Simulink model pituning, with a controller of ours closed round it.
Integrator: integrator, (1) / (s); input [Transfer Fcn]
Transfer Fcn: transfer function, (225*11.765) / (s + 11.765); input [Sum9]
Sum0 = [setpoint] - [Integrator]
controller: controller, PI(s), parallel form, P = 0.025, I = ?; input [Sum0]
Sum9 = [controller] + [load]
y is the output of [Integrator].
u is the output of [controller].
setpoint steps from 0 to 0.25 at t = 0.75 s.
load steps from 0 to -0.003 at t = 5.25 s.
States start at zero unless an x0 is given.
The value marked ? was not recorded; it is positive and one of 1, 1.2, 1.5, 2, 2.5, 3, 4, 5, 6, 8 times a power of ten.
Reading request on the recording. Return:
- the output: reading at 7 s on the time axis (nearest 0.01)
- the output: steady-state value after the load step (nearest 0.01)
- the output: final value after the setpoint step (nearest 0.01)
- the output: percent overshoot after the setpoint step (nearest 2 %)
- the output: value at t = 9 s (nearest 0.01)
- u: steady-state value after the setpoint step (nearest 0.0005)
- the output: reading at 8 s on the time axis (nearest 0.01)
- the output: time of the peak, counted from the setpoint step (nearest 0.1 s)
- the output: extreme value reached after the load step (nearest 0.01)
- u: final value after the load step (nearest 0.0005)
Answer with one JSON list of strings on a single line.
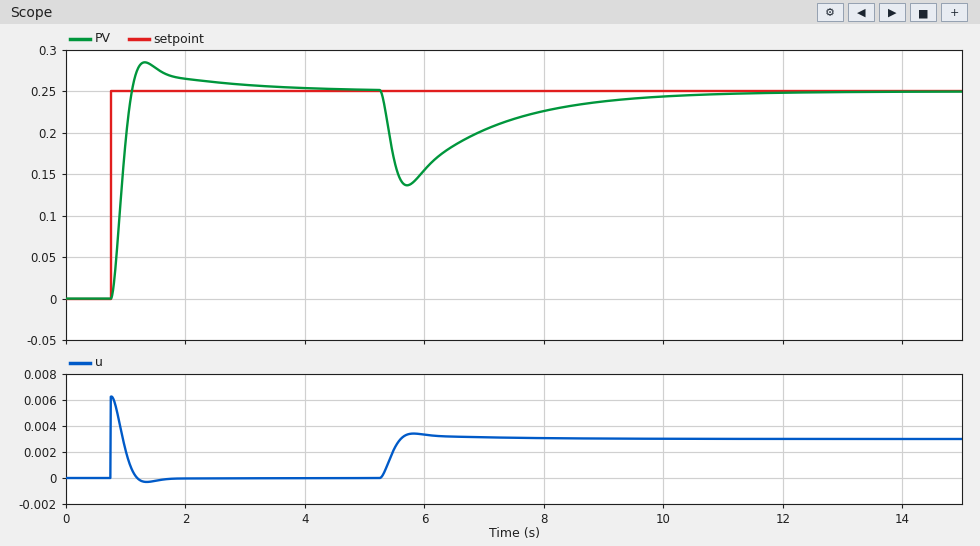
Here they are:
["0.20", "0.25", "0.25", "14 %", "0.24", "0.0000", "0.23", "0.6 s", "0.14", "0.0030"]
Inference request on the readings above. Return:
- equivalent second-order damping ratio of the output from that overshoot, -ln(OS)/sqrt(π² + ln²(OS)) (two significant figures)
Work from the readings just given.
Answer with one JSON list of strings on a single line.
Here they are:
["0.53"]
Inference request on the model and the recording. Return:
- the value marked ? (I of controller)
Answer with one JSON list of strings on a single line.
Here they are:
["0.015"]
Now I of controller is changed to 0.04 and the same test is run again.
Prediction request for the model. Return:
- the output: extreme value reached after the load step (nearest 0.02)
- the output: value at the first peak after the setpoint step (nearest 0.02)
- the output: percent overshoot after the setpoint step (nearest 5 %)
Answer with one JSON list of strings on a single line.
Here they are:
["0.14", "0.32", "30 %"]
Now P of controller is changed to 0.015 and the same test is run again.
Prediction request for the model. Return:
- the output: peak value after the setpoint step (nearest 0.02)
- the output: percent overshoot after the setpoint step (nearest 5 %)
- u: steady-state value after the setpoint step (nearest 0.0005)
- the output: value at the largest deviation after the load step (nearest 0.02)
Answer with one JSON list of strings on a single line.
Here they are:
["0.30", "20 %", "0.0000", "0.08"]
